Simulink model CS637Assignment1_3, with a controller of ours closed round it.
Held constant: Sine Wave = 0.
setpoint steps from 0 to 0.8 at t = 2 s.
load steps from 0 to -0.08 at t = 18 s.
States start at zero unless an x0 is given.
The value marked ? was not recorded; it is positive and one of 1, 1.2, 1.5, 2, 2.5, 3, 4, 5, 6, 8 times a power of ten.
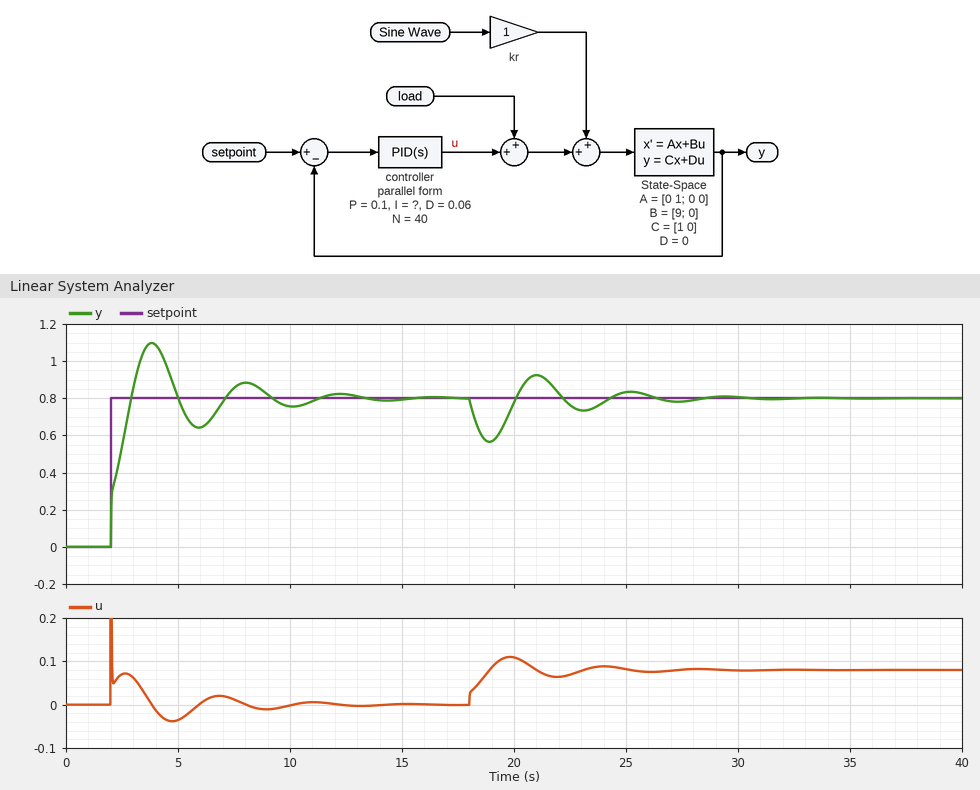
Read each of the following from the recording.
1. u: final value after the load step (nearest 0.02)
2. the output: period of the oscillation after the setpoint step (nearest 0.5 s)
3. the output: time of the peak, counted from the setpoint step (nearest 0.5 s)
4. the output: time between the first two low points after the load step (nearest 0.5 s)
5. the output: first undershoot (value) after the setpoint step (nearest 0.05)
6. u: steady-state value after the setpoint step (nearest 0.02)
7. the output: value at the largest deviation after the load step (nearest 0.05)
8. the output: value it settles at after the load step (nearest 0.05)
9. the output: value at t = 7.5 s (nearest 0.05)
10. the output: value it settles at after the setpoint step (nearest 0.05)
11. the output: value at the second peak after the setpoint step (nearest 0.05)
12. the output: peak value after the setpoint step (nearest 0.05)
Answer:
0.08
4.0 s
2.0 s
4.0 s
0.65
0.00
0.55
0.80
0.85
0.80
0.90
1.10
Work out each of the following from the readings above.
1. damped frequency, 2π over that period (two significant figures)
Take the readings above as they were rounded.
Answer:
1.6 rad/s
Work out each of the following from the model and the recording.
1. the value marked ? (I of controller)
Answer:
0.4
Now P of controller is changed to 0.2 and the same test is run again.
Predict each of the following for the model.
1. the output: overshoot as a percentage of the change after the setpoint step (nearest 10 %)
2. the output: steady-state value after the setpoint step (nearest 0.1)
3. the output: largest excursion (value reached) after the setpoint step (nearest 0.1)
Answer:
20 %
0.8
1.0
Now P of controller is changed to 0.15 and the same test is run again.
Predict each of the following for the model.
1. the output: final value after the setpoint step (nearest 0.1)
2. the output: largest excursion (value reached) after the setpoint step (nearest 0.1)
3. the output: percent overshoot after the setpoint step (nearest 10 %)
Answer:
0.8
1.0
30 %
